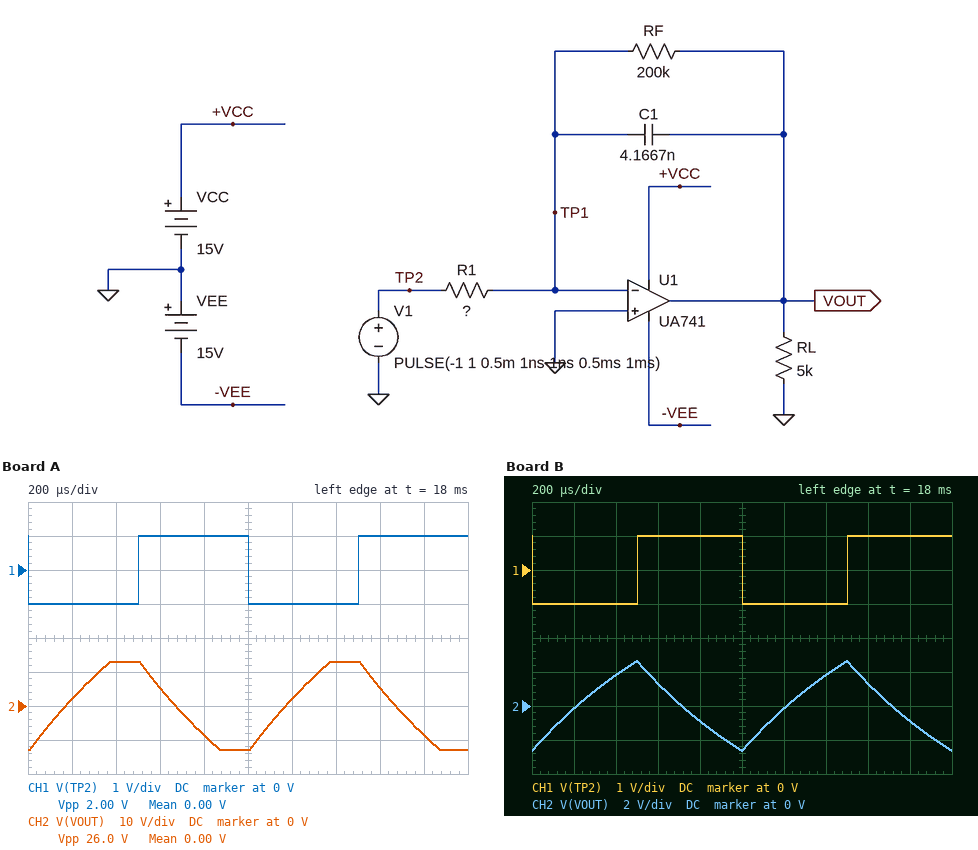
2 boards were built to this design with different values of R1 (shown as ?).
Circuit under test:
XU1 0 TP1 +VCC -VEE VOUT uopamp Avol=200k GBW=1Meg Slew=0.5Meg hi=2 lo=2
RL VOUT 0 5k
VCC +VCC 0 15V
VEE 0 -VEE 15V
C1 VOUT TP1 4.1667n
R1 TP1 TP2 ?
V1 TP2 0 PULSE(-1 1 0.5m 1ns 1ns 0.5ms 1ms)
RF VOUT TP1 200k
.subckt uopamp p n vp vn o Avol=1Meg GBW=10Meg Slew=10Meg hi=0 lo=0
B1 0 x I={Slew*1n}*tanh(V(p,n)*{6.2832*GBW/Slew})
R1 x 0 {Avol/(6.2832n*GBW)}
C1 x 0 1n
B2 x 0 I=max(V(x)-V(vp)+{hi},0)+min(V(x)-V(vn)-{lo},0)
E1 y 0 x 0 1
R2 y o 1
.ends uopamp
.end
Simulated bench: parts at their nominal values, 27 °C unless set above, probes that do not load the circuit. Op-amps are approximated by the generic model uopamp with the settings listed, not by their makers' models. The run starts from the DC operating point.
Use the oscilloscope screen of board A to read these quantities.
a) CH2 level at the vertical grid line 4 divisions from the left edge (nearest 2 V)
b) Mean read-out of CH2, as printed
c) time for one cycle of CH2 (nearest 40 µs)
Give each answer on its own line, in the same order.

-8 V
0.00 V
1.00 ms
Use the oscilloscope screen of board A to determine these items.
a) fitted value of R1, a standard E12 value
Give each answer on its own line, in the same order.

3.3 kΩ
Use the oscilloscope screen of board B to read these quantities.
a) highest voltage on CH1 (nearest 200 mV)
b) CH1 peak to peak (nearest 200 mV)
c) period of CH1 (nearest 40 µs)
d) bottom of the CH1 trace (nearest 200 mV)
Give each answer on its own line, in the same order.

1.0 V
2.0 V
1.00 ms
-1.0 V
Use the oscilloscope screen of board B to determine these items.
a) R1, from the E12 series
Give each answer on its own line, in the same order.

22 kΩ
